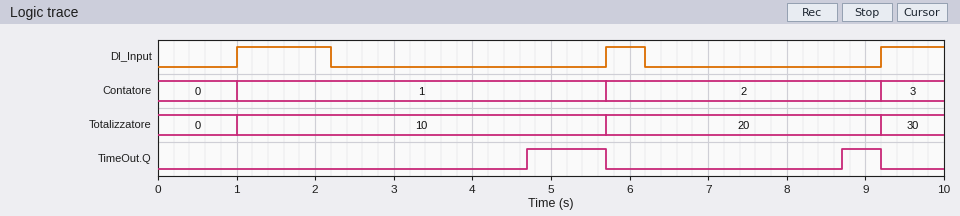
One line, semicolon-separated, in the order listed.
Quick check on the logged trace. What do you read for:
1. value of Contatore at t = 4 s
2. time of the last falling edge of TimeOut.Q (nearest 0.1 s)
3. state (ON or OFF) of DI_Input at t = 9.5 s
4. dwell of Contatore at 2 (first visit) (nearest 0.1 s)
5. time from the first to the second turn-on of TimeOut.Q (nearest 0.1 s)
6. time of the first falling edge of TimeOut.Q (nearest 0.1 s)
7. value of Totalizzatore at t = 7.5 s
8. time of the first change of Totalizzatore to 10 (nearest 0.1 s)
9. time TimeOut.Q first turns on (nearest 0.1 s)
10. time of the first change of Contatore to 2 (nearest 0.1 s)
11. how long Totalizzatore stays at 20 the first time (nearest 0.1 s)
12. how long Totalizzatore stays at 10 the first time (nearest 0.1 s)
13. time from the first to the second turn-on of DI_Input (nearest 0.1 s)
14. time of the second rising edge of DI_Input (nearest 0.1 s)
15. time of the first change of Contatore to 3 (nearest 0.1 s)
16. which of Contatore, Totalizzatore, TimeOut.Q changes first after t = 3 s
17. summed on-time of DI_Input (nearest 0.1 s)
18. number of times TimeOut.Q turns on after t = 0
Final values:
1; 9.2 s; ON; 3.5 s; 4.0 s; 5.7 s; 20; 1.0 s; 4.7 s; 5.7 s; 3.5 s; 4.7 s; 4.7 s; 5.7 s; 9.2 s; TimeOut.Q; 2.5 s; 2
